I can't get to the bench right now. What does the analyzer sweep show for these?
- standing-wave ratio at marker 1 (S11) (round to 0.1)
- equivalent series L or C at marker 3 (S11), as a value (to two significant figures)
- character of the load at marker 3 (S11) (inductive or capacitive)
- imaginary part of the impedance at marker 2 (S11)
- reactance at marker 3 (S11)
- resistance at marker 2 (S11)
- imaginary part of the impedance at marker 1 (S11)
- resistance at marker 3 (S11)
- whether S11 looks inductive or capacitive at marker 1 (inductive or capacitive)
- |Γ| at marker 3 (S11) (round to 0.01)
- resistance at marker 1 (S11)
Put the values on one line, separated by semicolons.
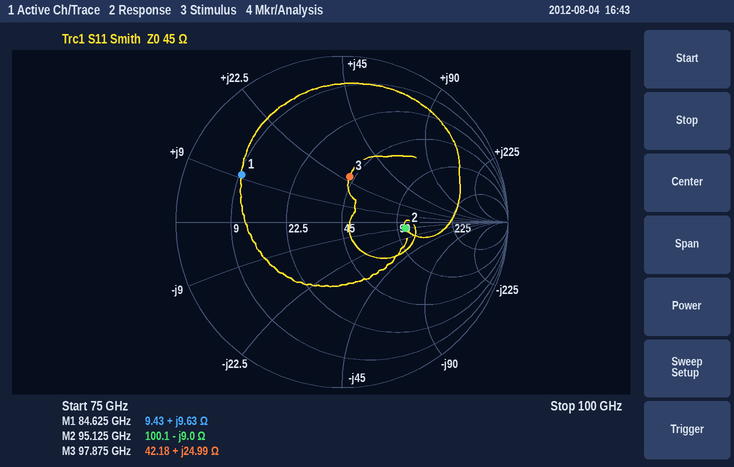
5.0; 41 pH; inductive; -9.0 Ω; +24.99 Ω; 100.1 Ω; +9.63 Ω; 42.18 Ω; inductive; 0.28; 9.43 Ω
